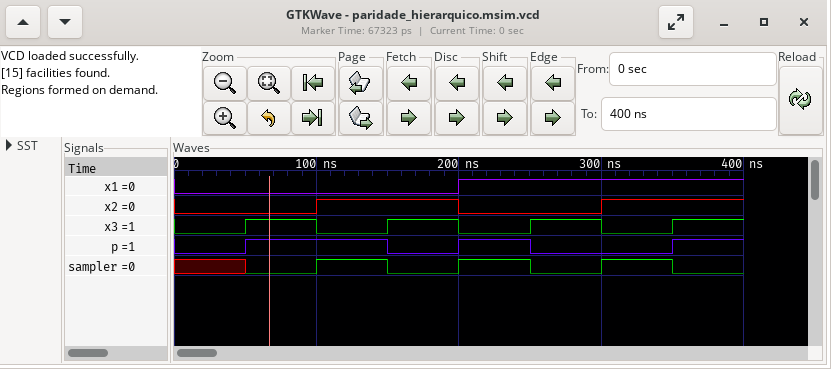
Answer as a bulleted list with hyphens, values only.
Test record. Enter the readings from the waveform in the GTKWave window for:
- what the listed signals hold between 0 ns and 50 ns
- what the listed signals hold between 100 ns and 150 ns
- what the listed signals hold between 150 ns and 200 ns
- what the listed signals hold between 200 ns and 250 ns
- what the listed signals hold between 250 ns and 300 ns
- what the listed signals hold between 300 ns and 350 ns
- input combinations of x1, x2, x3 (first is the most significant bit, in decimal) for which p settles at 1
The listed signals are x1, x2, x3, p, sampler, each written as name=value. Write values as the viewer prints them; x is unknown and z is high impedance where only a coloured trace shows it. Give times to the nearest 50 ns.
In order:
- x1=0, x2=0, x3=0, p=0, sampler=x
- x1=0, x2=1, x3=0, p=1, sampler=1
- x1=0, x2=1, x3=1, p=0, sampler=0
- x1=1, x2=0, x3=0, p=1, sampler=1
- x1=1, x2=0, x3=1, p=0, sampler=0
- x1=1, x2=1, x3=0, p=0, sampler=1
- 1, 2, 4, 7
